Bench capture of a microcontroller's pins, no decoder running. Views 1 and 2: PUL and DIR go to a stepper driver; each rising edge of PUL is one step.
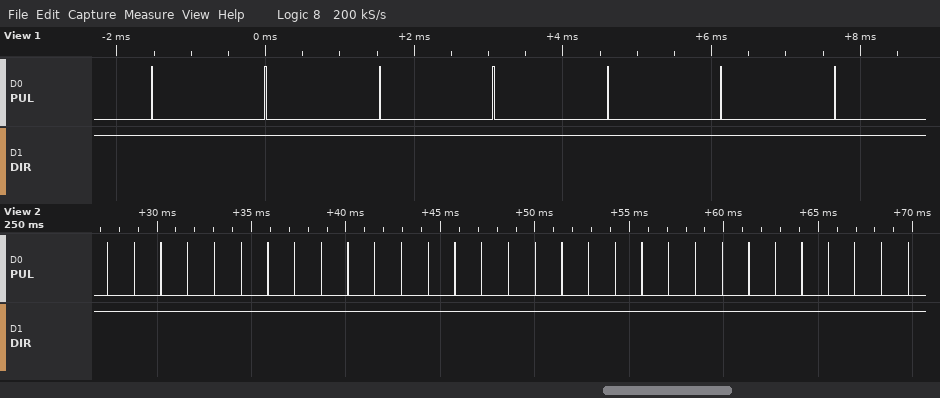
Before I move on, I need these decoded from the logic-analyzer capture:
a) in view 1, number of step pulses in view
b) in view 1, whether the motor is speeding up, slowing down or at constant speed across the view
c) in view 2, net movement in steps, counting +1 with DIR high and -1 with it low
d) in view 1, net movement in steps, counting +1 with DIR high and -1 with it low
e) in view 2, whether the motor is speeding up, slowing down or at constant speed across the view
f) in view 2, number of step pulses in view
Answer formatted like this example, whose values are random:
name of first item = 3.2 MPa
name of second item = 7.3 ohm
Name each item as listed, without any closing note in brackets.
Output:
in view 1, number of step pulses in view = 7
in view 1, whether the motor is speeding up, slowing down or at constant speed across the view = constant speed
in view 2, net movement in steps, counting +1 with DIR high and -1 with it low = +31
in view 1, net movement in steps, counting +1 with DIR high and -1 with it low = +7
in view 2, whether the motor is speeding up, slowing down or at constant speed across the view = constant speed
in view 2, number of step pulses in view = 31
